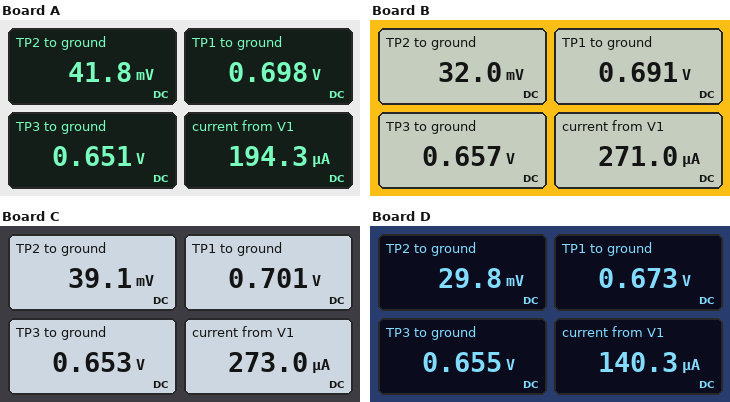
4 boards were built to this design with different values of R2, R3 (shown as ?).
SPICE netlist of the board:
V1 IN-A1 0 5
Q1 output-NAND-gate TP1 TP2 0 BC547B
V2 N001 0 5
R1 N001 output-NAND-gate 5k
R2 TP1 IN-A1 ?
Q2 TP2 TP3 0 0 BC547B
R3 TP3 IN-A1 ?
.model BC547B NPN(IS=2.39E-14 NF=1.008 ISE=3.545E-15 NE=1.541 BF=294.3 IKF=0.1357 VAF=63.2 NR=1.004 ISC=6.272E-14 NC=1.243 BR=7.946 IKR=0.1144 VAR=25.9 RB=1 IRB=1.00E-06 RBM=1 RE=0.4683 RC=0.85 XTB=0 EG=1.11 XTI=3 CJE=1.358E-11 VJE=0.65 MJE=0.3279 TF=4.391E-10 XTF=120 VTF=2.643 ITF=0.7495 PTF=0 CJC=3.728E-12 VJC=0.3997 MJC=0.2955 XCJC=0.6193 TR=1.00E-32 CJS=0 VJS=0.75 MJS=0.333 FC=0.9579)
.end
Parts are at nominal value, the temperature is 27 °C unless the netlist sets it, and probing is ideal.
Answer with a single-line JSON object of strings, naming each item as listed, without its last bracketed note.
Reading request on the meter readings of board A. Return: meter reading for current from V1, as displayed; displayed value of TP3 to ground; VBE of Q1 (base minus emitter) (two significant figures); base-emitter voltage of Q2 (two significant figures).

{"meter reading for current from V1, as displayed": "194.3 µA", "displayed value of TP3 to ground": "0.651 V", "VBE of Q1 (base minus emitter)": "660 mV", "base-emitter voltage of Q2": "650 mV"}
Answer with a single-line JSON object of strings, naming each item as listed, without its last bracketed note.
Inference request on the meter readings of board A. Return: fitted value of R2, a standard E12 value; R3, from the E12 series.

{"fitted value of R2, a standard E12 value": "33 kΩ", "R3, from the E12 series": "68 kΩ"}
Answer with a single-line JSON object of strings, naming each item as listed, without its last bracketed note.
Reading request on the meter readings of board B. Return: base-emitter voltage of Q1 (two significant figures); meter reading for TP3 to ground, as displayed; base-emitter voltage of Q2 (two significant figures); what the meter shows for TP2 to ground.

{"base-emitter voltage of Q1": "660 mV", "meter reading for TP3 to ground, as displayed": "0.657 V", "base-emitter voltage of Q2": "660 mV", "what the meter shows for TP2 to ground": "32.0 mV"}
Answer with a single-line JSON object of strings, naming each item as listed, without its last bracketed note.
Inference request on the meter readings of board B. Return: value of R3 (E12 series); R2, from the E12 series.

{"value of R3": "39 kΩ", "R2, from the E12 series": "27 kΩ"}
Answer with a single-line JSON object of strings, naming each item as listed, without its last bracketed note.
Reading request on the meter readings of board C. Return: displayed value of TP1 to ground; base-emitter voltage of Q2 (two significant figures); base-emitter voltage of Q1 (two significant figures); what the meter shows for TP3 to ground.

{"displayed value of TP1 to ground": "0.701 V", "base-emitter voltage of Q2": "650 mV", "base-emitter voltage of Q1": "660 mV", "what the meter shows for TP3 to ground": "0.653 V"}
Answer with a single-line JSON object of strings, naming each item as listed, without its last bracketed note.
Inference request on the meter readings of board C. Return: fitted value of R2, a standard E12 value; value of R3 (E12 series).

{"fitted value of R2, a standard E12 value": "22 kΩ", "value of R3": "56 kΩ"}
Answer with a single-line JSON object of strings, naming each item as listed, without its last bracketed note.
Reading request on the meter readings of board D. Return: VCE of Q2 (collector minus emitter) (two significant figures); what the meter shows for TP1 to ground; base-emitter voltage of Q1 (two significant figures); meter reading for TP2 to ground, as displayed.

{"VCE of Q2 (collector minus emitter)": "30 mV", "what the meter shows for TP1 to ground": "0.673 V", "base-emitter voltage of Q1": "640 mV", "meter reading for TP2 to ground, as displayed": "29.8 mV"}
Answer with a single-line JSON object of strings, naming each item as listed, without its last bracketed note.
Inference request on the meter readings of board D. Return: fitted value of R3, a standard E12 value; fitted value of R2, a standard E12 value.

{"fitted value of R3, a standard E12 value": "39 kΩ", "fitted value of R2, a standard E12 value": "150 kΩ"}
